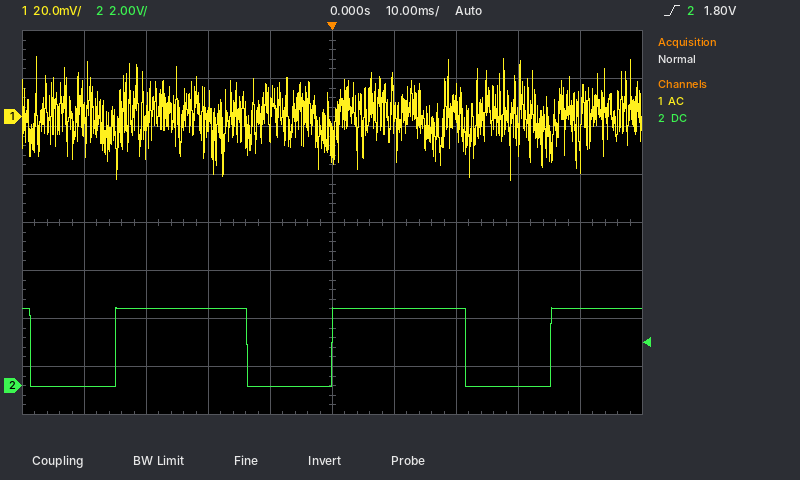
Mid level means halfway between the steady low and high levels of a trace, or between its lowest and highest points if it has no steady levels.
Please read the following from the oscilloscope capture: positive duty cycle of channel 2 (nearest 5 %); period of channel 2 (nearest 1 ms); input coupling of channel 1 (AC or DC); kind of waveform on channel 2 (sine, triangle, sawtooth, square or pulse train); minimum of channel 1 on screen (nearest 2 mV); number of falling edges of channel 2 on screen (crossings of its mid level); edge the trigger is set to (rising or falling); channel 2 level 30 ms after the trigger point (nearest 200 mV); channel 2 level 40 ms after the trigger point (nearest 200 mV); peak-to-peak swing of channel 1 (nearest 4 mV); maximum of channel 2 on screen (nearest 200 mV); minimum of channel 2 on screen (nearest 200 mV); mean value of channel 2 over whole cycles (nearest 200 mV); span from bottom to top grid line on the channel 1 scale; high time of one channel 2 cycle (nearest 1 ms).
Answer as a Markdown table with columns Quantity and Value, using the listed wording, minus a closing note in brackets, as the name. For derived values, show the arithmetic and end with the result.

| Quantity | Value |
|---|---|
| positive duty cycle of channel 2 | 21 ms / 35 ms ≈ 60 % |
| period of channel 2 | 35 ms |
| input coupling of channel 1 | AC |
| kind of waveform on channel 2 | pulse train |
| minimum of channel 1 on screen | -26 mV |
| number of falling edges of channel 2 on screen | 3 |
| edge the trigger is set to | rising |
| channel 2 level 30 ms after the trigger point | 0.0 V |
| channel 2 level 40 ms after the trigger point | 3.2 V |
| peak-to-peak swing of channel 1 | 52 mV |
| maximum of channel 2 on screen | 3.2 V |
| minimum of channel 2 on screen | 0.0 V |
| mean value of channel 2 over whole cycles | 0.0 V + 0.6 × (3.2 V − (0.0 V)) ≈ 1.92 V, so 2.0 V to the nearest 200 mV |
| span from bottom to top grid line on the channel 1 scale | 160 mV |
| high time of one channel 2 cycle | 21 ms |
